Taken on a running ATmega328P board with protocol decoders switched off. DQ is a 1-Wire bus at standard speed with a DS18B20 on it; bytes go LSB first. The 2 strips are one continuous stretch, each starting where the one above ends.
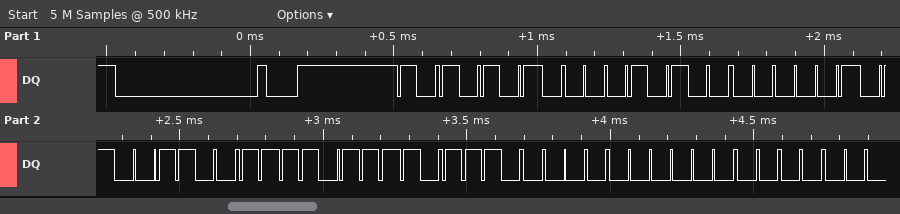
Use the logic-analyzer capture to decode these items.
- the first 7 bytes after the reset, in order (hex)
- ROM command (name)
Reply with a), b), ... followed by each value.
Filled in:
a) 55 28 A0 CC 7B 07 00
b) Match ROM
